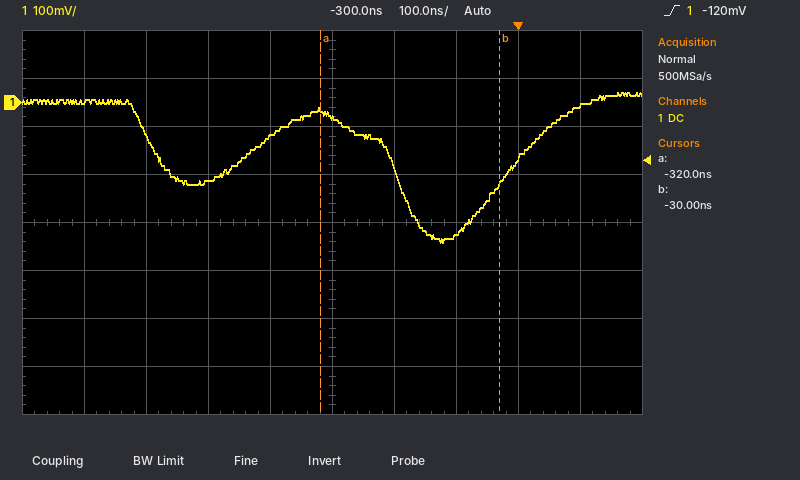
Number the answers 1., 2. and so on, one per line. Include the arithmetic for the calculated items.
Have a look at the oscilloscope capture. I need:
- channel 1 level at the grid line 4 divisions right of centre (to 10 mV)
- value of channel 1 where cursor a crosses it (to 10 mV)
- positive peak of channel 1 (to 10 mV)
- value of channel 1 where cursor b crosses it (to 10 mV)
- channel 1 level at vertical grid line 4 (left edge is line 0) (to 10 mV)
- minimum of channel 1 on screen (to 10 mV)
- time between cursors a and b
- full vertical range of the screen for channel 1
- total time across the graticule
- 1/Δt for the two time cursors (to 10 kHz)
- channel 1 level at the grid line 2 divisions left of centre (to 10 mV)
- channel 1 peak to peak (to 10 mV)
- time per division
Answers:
1. -10 mV
2. -20 mV
3. 20 mV
4. -170 mV
5. -70 mV
6. -290 mV
7. -30 ns − (-320 ns) = 290 ns
8. 800 mV
9. 1 µs
10. 1 / 290 ns ≈ 3.45 MHz
11. -160 mV
12. 20 mV − (-290 mV) = 310 mV
13. 100 ns
